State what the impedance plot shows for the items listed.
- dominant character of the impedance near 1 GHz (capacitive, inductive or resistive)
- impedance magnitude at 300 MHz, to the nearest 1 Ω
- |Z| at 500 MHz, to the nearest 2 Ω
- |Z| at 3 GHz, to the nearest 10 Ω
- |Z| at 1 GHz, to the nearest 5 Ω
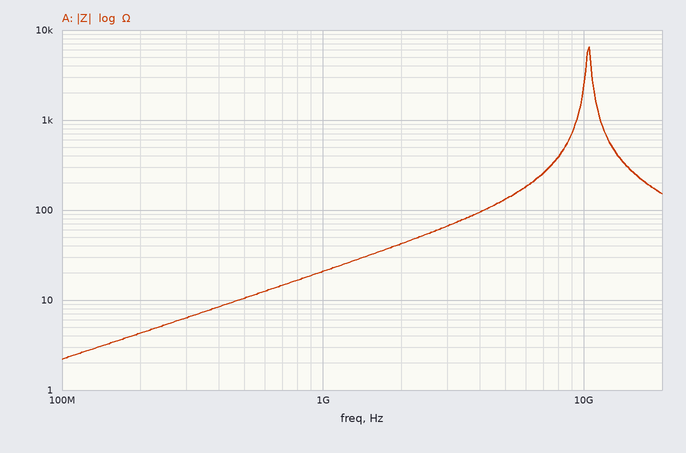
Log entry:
inductive
6 Ω
10 Ω
70 Ω
20 Ω
